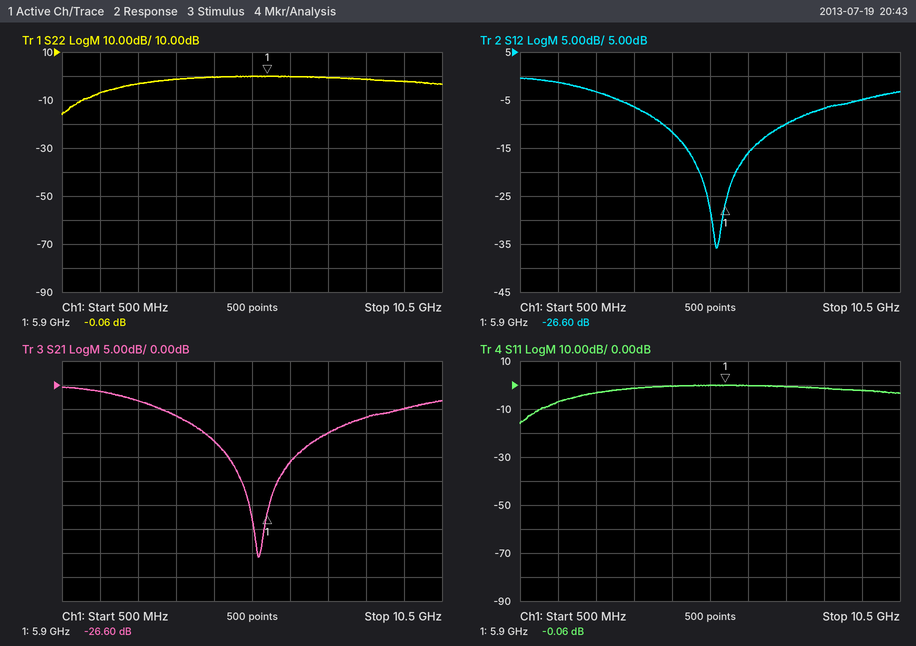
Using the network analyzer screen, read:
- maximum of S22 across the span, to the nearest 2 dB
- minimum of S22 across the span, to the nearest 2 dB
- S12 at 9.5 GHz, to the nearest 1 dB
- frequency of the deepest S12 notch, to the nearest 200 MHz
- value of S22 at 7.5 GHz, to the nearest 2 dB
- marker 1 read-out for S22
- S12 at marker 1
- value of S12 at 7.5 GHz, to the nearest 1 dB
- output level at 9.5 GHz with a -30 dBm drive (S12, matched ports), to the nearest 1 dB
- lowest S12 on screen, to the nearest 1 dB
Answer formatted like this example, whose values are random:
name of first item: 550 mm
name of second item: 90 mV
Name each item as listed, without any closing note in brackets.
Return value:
maximum of S22 across the span, to the nearest 2 dB: 0 dB
minimum of S22 across the span, to the nearest 2 dB: -16 dB
S12 at 9.5 GHz, to the nearest 1 dB: -5 dB
frequency of the deepest S12 notch, to the nearest 200 MHz: 5.6 GHz
value of S22 at 7.5 GHz, to the nearest 2 dB: 0 dB
marker 1 read-out for S22: -0.06 dB
S12 at marker 1: -26.60 dB
value of S12 at 7.5 GHz, to the nearest 1 dB: -10 dB
output level at 9.5 GHz with a -30 dBm drive (S12, matched ports), to the nearest 1 dB: -35 dBm
lowest S12 on screen, to the nearest 1 dB: -36 dB
